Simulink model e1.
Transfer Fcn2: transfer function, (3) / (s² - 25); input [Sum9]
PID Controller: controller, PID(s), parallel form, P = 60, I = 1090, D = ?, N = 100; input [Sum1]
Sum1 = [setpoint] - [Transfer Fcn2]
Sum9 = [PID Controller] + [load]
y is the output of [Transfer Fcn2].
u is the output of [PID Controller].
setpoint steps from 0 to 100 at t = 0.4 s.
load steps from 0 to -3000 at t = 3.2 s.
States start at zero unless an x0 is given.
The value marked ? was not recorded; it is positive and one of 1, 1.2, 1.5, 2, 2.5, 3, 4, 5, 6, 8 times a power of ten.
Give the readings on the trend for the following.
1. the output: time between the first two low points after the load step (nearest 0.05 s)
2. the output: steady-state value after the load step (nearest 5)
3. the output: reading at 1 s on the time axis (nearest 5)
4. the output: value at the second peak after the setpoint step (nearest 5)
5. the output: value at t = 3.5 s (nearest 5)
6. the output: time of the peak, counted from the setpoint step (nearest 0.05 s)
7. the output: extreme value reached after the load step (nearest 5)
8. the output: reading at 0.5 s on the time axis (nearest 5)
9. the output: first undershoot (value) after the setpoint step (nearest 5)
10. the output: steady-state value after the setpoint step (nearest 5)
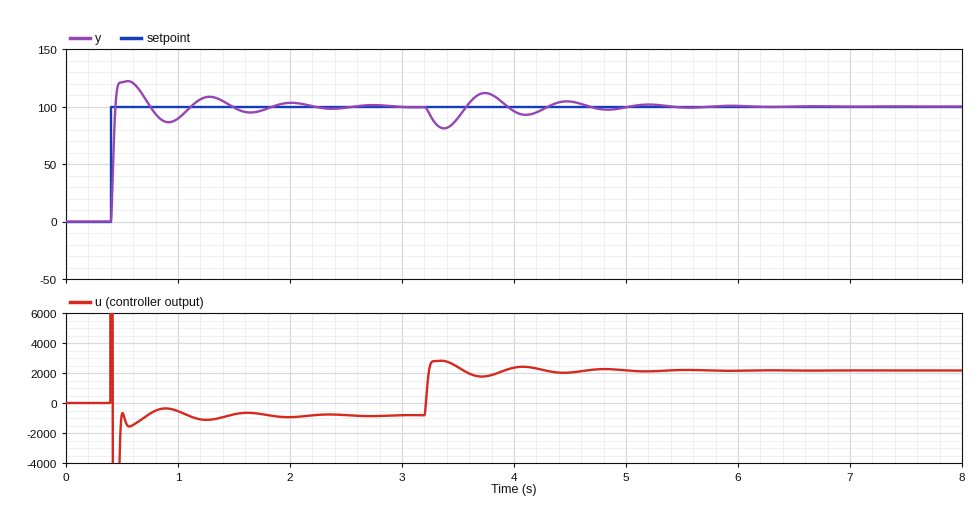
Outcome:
0.75 s
100
90
110
90
0.15 s
80
120
85
100
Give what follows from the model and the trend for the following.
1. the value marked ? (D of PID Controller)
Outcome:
15
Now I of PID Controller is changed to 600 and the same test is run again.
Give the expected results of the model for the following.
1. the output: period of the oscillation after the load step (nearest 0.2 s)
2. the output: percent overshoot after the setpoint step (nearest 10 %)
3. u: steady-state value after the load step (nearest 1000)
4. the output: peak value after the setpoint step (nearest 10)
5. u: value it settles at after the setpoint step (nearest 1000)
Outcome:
1.0 s
20 %
2000
120
-1000
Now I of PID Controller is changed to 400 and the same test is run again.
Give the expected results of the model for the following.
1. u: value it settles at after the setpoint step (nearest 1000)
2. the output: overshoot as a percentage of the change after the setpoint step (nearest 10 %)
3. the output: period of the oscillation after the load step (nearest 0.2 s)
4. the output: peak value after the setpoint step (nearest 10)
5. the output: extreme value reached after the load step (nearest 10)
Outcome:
-1000
20 %
1.2 s
120
70
